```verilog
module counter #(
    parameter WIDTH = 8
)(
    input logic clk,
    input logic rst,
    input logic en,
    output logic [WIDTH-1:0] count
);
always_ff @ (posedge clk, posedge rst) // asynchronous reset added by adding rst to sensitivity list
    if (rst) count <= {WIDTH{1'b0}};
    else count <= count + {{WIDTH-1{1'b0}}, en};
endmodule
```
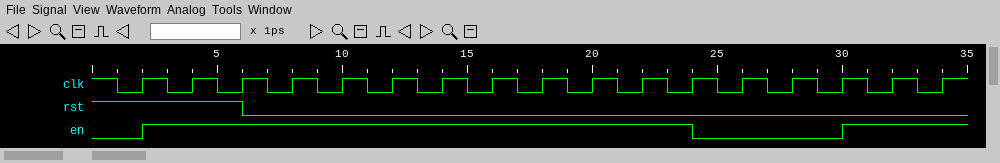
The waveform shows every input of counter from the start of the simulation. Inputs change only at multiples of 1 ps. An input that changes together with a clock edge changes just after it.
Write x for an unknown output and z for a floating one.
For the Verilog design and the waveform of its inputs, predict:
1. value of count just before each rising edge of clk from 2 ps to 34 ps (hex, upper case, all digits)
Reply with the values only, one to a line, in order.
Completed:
00, 00, 00, 00, 01, 02, 03, 04, 05, 06, 07, 08, 09, 09, 09, 09, 0A
